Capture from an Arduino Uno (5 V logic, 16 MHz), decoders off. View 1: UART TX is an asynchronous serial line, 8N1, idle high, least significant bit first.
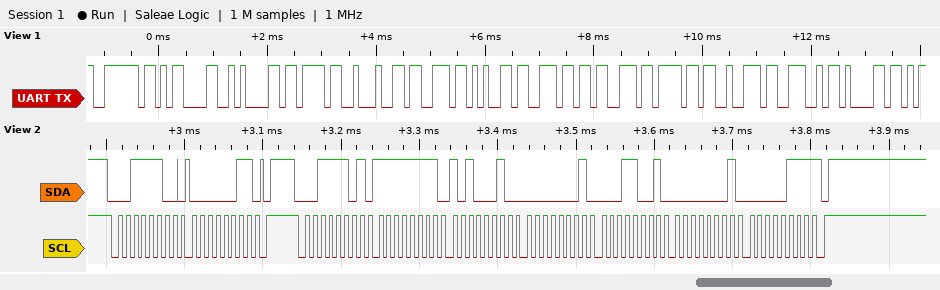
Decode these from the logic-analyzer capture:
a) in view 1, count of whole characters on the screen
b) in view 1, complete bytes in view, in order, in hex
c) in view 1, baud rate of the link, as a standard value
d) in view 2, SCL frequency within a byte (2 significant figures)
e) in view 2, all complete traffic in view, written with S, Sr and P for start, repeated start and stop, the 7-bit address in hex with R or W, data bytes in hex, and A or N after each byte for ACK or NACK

13
7E 0D 0A 7B 22 73 65 6E 73 6F 72 4E 61
9600 baud
100 kHz
S 1EW A 03 A P S 1ER A FF A A2 A 01 A 19 A 01 A 07 N P
